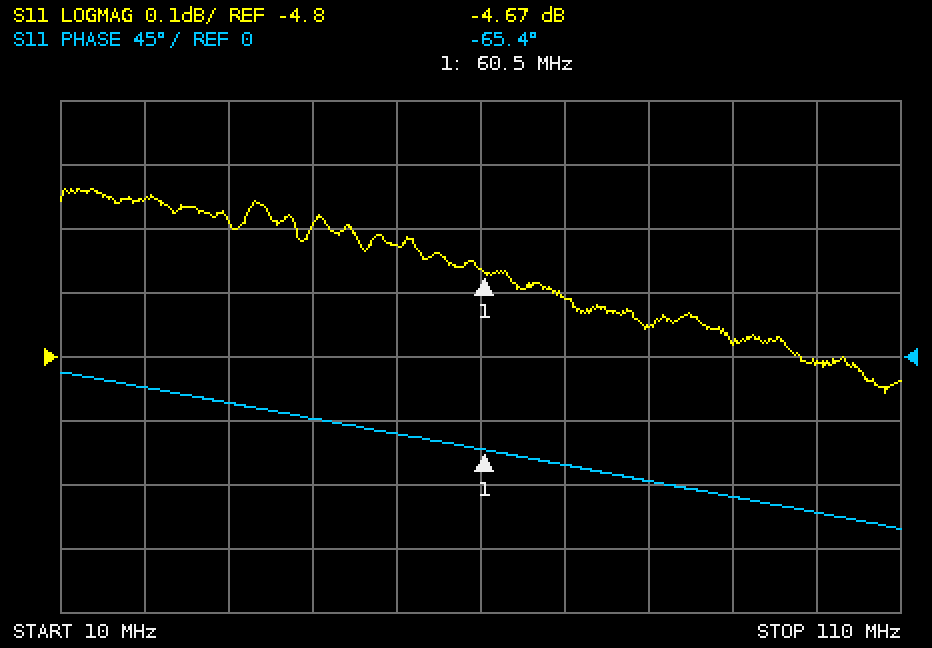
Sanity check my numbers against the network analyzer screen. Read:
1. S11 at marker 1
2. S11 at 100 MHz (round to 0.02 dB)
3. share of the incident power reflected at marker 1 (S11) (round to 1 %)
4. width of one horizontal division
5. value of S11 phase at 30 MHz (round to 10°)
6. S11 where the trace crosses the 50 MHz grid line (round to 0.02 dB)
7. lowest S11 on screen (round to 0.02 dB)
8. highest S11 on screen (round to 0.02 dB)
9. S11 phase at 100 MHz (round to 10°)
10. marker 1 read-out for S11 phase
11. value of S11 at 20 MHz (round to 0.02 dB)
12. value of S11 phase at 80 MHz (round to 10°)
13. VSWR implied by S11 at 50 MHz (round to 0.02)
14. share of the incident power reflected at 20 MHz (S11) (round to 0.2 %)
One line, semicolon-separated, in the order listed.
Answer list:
-4.67 dB; -4.80 dB; 34 %; 10 MHz; -30°; -4.62 dB; -4.86 dB; -4.54 dB; -110°; -65.4°; -4.56 dB; -90°; 3.84; 35.0 %
